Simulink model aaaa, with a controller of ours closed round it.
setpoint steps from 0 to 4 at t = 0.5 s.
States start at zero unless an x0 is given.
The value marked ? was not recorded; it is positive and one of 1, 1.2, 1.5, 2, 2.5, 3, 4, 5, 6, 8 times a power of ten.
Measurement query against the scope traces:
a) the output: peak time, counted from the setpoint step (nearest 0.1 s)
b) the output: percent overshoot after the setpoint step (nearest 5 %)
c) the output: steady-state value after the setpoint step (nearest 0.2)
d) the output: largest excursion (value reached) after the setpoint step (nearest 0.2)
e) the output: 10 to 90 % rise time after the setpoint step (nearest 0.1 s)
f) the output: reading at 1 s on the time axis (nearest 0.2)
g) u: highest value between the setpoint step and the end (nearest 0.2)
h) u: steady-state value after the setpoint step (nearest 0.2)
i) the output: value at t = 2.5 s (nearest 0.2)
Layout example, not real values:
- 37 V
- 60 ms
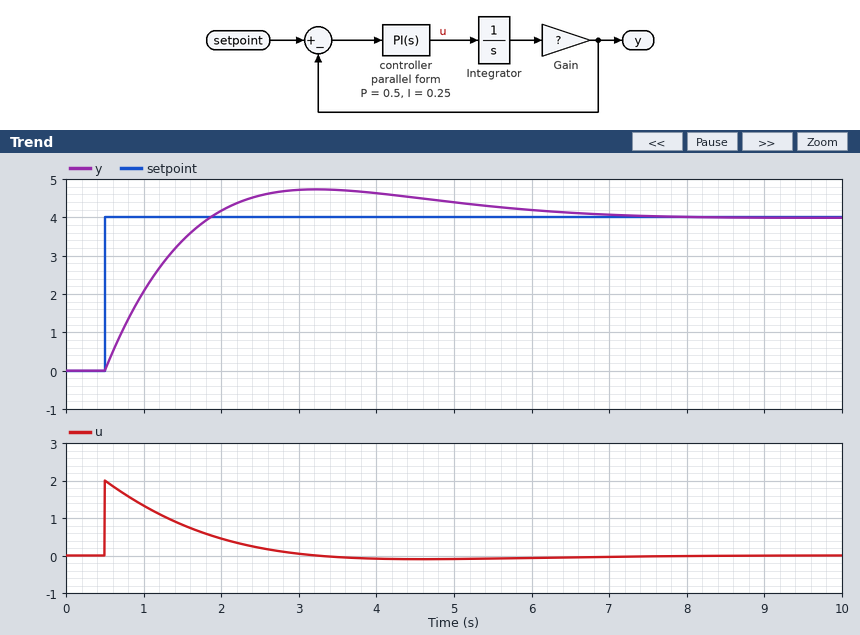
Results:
- 2.7 s
- 20 %
- 4.0
- 4.8
- 1.0 s
- 2.0
- 2.0
- 0.0
- 4.6
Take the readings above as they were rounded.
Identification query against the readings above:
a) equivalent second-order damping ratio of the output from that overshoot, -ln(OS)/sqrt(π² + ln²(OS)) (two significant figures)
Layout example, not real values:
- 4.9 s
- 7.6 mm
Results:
- 0.46
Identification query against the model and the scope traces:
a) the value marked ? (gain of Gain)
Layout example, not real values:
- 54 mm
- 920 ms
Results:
- 2.5
